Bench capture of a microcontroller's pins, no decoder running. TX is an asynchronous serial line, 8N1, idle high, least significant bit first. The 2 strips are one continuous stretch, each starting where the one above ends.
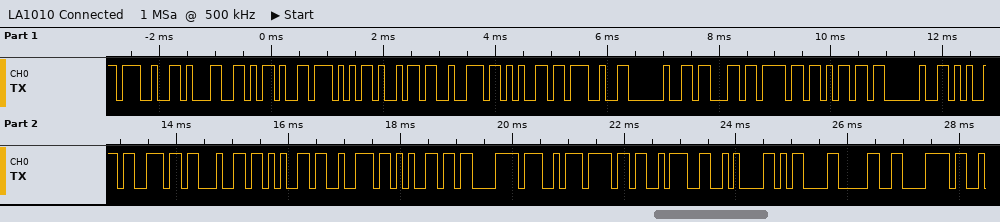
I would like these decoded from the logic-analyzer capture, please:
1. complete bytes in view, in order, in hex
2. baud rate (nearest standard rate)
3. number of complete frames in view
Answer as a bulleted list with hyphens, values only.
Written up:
- 27 31 2D 57 69 72 65 27 20 63 6F 6D 20 65 6E 64 65 72 65 C3 A7 6F 3A 0A 0D 30 78
- 9600 baud
- 27
